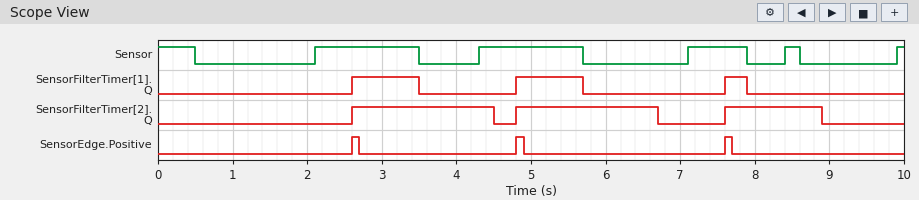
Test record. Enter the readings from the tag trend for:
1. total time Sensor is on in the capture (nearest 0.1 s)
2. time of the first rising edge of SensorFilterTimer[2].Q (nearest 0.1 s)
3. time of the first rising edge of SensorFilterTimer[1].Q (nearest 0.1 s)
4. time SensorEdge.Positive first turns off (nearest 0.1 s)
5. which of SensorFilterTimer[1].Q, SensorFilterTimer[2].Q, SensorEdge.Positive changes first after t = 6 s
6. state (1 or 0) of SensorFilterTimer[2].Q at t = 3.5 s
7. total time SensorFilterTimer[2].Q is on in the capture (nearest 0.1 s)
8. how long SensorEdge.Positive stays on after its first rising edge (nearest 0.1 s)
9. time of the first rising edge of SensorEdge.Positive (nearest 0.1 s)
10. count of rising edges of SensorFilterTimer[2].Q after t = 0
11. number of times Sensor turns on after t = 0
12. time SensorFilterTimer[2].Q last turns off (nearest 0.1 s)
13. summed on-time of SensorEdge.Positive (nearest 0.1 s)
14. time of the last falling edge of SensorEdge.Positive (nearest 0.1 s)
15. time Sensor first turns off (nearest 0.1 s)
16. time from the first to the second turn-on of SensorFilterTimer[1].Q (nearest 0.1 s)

4.4 s
2.6 s
2.6 s
2.7 s
SensorFilterTimer[2].Q
1
5.1 s
0.1 s
2.6 s
3
5
8.9 s
0.3 s
7.7 s
0.5 s
2.2 s
